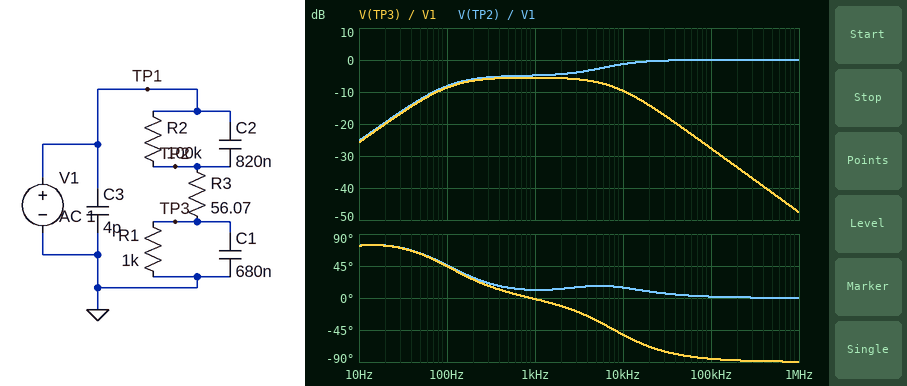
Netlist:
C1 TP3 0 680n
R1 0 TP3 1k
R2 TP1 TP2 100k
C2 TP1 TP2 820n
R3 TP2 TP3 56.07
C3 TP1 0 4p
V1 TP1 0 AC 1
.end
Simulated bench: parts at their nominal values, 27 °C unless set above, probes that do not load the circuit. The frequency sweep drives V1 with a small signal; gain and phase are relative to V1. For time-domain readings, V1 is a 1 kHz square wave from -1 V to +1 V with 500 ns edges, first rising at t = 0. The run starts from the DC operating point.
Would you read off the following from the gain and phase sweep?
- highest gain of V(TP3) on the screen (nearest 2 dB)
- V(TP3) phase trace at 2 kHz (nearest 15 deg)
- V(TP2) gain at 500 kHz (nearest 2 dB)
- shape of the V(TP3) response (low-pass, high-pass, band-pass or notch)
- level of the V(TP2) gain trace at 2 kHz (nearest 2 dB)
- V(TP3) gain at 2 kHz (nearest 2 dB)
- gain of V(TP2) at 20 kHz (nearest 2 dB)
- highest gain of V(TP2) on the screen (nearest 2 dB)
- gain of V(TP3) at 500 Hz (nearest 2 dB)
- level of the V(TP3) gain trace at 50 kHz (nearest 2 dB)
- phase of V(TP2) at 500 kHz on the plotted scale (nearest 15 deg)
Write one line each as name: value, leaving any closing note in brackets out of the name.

highest gain of V(TP3) on the screen: -6 dB
V(TP3) phase trace at 2 kHz: -15 deg
V(TP2) gain at 500 kHz: 0 dB
shape of the V(TP3) response: band-pass
level of the V(TP2) gain trace at 2 kHz: -4 dB
V(TP3) gain at 2 kHz: -6 dB
gain of V(TP2) at 20 kHz: 0 dB
highest gain of V(TP2) on the screen: 0 dB
gain of V(TP3) at 500 Hz: -6 dB
level of the V(TP3) gain trace at 50 kHz: -22 dB
phase of V(TP2) at 500 kHz on the plotted scale: 0 deg
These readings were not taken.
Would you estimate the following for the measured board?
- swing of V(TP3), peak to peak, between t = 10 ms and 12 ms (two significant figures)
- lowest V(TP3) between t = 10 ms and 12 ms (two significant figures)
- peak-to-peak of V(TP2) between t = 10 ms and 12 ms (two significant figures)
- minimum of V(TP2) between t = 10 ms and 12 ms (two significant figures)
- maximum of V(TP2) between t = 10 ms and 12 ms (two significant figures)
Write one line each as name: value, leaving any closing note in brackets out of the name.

swing of V(TP3), peak to peak, between t = 10 ms and 12 ms: 1.2 V
lowest V(TP3) between t = 10 ms and 12 ms: -580 mV
peak-to-peak of V(TP2) between t = 10 ms and 12 ms: 3.0 V
minimum of V(TP2) between t = 10 ms and 12 ms: -1.5 V
maximum of V(TP2) between t = 10 ms and 12 ms: 1.5 V
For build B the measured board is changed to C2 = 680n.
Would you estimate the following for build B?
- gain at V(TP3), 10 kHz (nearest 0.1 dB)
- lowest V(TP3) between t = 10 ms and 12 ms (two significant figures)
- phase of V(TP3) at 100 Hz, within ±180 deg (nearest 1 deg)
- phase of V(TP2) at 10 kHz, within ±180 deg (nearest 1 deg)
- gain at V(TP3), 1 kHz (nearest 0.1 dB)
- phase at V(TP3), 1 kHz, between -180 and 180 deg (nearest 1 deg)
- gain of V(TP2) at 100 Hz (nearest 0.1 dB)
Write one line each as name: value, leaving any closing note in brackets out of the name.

gain at V(TP3), 10 kHz: -9.9 dB
lowest V(TP3) between t = 10 ms and 12 ms: -540 mV
phase of V(TP3) at 100 Hz, within ±180 deg: 47 deg
phase of V(TP2) at 10 kHz, within ±180 deg: 17 deg
gain at V(TP3), 1 kHz: -6.3 dB
phase at V(TP3), 1 kHz, between -180 and 180 deg: 0 deg
gain of V(TP2) at 100 Hz: -9.4 dB
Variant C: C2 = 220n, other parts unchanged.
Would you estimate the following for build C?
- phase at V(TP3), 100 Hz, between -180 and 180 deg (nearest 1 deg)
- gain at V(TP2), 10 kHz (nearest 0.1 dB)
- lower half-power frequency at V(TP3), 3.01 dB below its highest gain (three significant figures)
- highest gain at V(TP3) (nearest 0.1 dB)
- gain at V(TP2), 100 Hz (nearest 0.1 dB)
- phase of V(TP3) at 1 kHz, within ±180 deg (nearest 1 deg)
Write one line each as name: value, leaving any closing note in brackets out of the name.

phase at V(TP3), 100 Hz, between -180 and 180 deg: 56 deg
gain at V(TP2), 10 kHz: -5.2 dB
lower half-power frequency at V(TP3), 3.01 dB below its highest gain: 174 Hz
highest gain at V(TP3): -12.4 dB
gain at V(TP2), 100 Hz: -18.0 dB
phase of V(TP3) at 1 kHz, within ±180 deg: 6 deg
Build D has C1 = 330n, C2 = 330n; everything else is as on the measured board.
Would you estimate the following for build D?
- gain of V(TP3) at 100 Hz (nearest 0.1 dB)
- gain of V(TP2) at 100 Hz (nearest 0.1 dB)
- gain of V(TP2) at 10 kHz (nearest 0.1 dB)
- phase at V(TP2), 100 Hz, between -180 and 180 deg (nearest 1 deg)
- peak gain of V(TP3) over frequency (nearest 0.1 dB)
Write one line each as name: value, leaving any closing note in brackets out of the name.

gain of V(TP3) at 100 Hz: -14.4 dB
gain of V(TP2) at 100 Hz: -14.0 dB
gain of V(TP2) at 10 kHz: -3.5 dB
phase at V(TP2), 100 Hz, between -180 and 180 deg: 65 deg
peak gain of V(TP3) over frequency: -6.3 dB
